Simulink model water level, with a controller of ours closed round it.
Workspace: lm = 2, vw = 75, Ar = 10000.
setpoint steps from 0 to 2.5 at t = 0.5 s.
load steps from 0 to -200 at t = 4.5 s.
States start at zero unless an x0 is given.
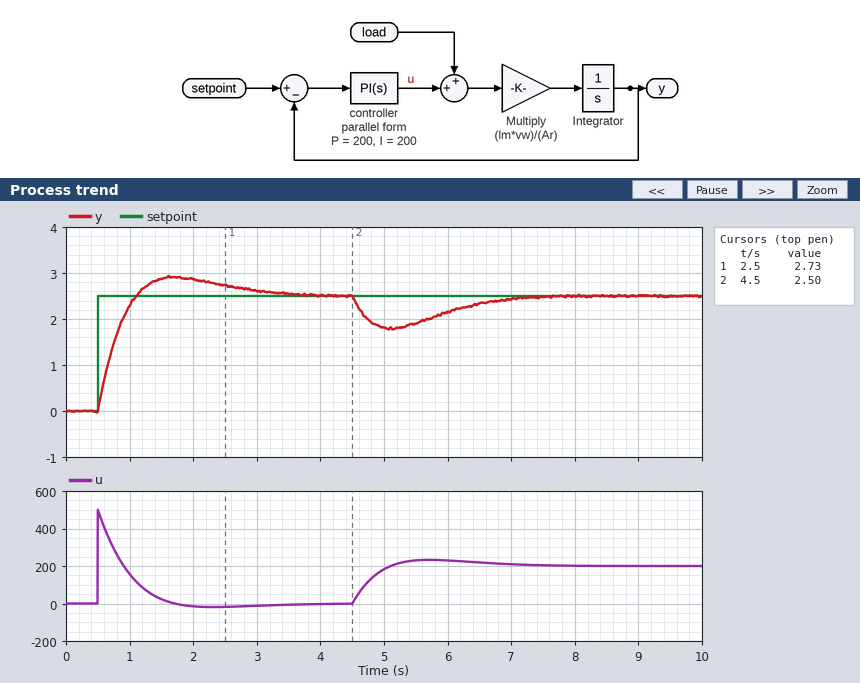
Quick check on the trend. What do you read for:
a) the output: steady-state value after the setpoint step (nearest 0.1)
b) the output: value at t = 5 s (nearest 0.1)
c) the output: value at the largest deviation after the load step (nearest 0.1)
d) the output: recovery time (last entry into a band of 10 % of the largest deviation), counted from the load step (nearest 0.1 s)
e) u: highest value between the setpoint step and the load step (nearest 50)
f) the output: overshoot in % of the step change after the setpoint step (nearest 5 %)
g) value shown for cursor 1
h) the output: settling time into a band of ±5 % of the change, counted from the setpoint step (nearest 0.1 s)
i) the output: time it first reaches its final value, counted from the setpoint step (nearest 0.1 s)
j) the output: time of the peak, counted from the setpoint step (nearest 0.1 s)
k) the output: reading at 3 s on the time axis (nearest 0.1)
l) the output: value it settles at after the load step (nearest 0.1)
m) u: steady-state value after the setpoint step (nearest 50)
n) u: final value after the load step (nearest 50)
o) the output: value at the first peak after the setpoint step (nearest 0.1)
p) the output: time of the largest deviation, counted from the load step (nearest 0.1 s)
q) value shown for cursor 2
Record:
2.5
1.8
1.8
2.5 s
500
15 %
2.73
2.5 s
0.6 s
1.2 s
2.6
2.5
0
200
2.9
0.6 s
2.50
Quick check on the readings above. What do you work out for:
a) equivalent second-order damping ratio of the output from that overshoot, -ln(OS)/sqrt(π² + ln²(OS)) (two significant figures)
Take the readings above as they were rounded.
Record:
0.52
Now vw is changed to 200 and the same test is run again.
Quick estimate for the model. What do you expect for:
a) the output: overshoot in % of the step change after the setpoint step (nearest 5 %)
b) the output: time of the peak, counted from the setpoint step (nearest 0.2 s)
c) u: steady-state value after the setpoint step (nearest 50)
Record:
10 %
0.6 s
0
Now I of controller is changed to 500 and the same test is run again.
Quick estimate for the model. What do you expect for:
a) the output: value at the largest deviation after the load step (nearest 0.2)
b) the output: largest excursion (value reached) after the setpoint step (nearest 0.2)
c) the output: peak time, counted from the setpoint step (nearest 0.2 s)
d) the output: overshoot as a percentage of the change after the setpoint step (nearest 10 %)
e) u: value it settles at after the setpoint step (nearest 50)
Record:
2.0
3.2
0.8 s
30 %
0
